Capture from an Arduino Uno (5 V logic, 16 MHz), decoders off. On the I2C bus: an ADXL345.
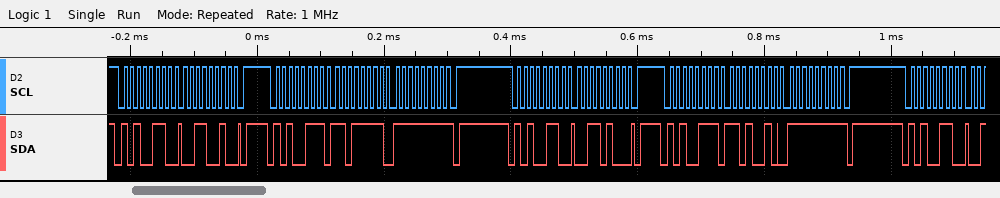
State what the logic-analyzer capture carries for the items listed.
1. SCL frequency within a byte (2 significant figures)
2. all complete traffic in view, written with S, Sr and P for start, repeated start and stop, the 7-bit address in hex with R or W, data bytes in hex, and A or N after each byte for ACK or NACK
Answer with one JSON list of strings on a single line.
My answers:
["100 kHz", "S 53W A 32 A P S 53R A DF A FF N P S 53W A 34 A P S 53R A D2 A FF N P S 53W A"]
